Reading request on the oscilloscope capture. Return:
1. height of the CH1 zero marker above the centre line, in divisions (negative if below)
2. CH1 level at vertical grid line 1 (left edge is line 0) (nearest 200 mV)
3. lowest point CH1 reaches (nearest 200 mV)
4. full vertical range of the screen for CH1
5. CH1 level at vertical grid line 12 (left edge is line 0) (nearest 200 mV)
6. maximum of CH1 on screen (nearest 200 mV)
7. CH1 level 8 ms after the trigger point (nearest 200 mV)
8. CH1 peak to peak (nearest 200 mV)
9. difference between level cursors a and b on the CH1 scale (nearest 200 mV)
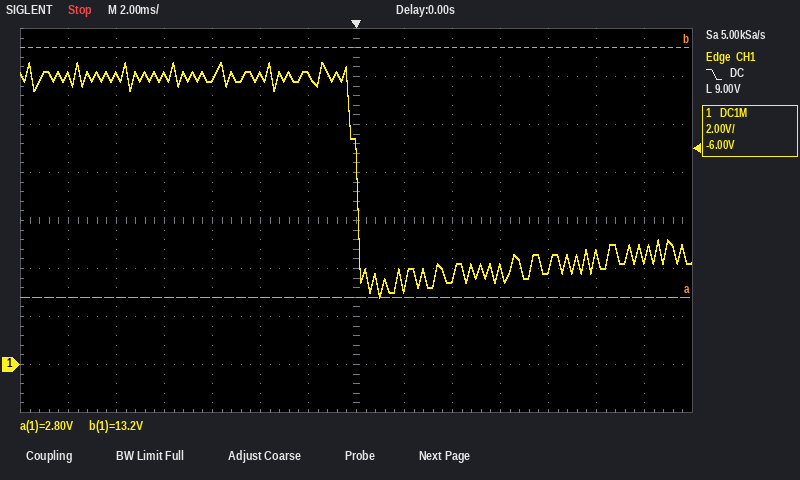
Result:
-3.0 div
12.0 V
2.8 V
16 V
4.6 V
12.6 V
4.0 V
9.8 V
10.4 V
